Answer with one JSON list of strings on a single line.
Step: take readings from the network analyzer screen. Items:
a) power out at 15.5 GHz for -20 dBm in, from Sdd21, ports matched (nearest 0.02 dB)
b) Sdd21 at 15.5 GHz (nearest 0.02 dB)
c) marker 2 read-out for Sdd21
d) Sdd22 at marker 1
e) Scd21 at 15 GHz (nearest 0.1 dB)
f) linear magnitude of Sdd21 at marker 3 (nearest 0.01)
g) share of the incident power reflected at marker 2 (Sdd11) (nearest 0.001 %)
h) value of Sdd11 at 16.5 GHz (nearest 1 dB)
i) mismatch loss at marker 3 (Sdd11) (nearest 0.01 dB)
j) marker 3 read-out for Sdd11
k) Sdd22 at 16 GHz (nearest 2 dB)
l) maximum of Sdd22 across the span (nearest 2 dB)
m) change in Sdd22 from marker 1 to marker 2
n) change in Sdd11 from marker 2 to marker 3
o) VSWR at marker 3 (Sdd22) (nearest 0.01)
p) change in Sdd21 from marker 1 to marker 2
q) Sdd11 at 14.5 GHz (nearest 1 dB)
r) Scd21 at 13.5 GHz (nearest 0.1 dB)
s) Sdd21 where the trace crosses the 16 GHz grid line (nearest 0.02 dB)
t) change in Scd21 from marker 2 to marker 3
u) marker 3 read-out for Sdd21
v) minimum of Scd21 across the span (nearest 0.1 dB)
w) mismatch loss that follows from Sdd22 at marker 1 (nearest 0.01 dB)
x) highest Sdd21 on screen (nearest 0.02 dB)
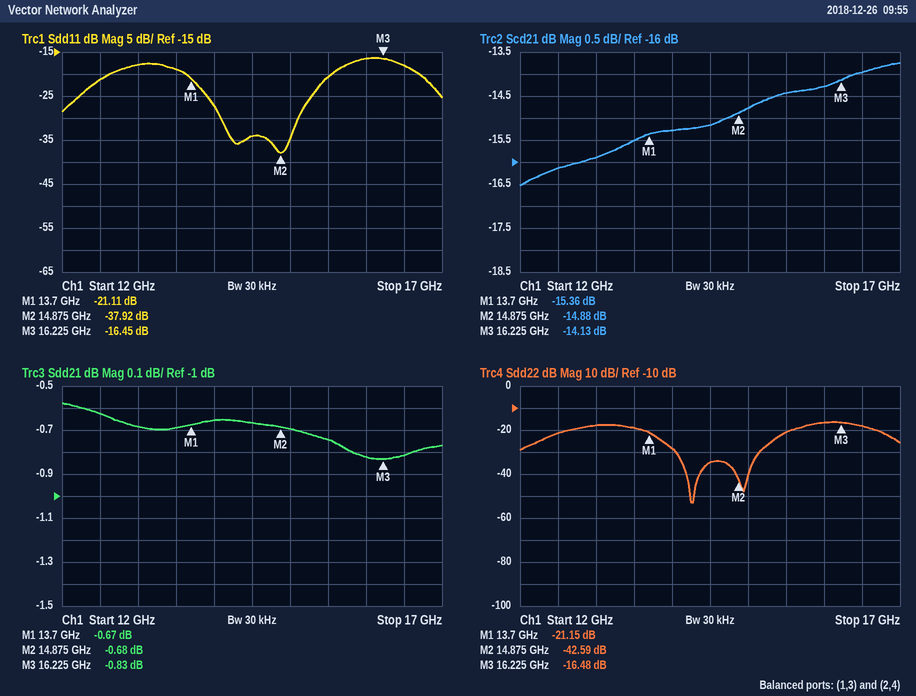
["-20.74 dBm", "-0.74 dB", "-0.68 dB", "-21.15 dB", "-14.8 dB", "0.91", "0.016 %", "-18 dB", "0.10 dB", "-16.45 dB", "-16 dB", "-16 dB", "-21.44 dB", "21.47 dB", "1.35", "-0.01 dB", "-34 dB", "-15.5 dB", "-0.82 dB", "0.75 dB", "-0.83 dB", "-16.5 dB", "0.03 dB", "-0.58 dB"]
